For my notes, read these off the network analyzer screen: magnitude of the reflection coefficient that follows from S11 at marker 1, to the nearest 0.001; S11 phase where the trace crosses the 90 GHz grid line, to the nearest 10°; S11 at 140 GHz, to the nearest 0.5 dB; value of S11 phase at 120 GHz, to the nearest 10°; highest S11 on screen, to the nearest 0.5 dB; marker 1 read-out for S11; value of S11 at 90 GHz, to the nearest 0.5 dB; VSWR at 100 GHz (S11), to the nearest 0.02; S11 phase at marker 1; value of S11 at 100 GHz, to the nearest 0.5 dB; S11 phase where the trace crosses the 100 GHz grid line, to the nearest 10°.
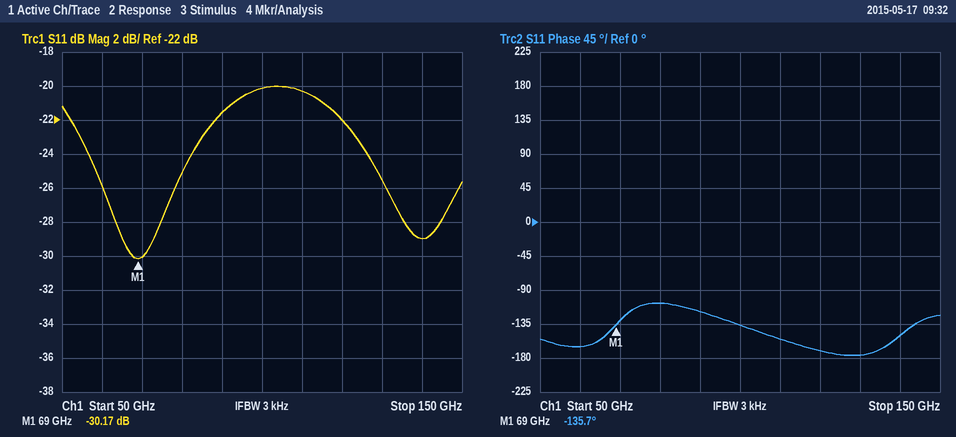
0.031
-120°
-29.0 dB
-170°
-20.0 dB
-30.17 dB
-21.5 dB
1.22
-135.7°
-20.0 dB
-140°
